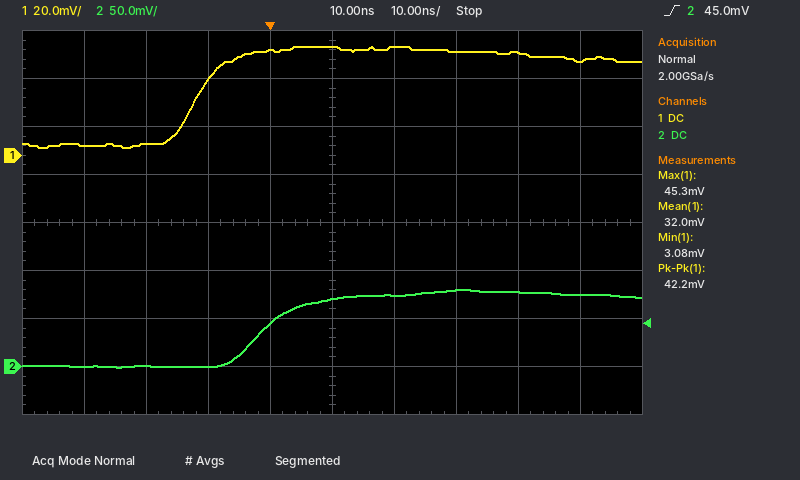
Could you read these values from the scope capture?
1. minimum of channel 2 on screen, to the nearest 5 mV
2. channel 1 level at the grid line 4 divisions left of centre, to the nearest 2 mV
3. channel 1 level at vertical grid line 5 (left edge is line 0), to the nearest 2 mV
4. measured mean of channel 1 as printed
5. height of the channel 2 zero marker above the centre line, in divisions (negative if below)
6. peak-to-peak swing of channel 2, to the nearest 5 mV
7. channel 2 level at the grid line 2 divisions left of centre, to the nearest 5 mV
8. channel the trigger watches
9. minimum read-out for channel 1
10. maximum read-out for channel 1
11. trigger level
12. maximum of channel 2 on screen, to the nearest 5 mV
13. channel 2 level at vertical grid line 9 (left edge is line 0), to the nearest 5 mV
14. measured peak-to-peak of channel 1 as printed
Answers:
0 mV
4 mV
46 mV
32.0 mV
-3.0 div
80 mV
0 mV
channel 2
3.08 mV
45.3 mV
45.0 mV
80 mV
75 mV
42.2 mV
